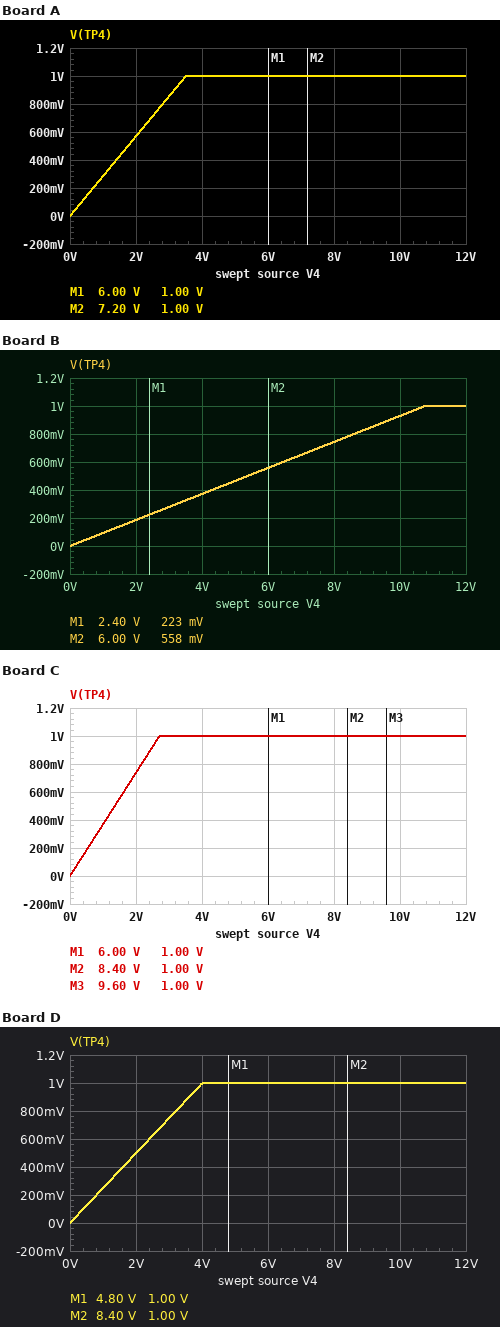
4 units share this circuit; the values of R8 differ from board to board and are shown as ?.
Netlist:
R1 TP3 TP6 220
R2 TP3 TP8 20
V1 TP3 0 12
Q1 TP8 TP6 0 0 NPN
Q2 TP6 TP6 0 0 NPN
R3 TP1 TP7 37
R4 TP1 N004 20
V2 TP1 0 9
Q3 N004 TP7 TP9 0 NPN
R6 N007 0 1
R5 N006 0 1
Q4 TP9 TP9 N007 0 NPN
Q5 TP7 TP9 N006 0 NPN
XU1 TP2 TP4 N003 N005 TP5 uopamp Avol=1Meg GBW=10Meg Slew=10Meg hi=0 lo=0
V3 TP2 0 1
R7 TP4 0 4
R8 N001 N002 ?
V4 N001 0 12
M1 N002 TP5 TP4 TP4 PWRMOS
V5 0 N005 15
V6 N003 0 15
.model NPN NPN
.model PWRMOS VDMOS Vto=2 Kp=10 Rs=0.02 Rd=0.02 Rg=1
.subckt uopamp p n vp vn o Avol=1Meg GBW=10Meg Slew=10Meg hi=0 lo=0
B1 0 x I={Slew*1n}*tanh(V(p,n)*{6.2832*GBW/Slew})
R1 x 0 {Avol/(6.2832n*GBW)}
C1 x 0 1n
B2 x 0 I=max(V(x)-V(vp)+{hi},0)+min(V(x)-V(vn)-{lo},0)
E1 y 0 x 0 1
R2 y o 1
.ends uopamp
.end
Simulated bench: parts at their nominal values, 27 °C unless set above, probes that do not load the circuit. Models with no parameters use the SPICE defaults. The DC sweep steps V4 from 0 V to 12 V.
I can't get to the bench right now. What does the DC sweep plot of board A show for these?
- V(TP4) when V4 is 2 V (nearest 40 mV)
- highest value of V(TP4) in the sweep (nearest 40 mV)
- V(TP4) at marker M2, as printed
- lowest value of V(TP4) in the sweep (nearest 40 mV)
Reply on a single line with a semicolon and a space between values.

560 mV; 1.00 V; 1.00 V; 0 V
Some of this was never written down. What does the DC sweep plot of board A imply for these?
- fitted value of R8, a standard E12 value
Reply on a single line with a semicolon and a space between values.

10 Ω
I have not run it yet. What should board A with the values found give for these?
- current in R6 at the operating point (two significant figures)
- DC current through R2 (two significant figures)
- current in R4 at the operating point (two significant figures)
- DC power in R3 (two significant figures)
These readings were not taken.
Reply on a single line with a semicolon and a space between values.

190 mA; 50 mA; 190 mA; 1.3 W
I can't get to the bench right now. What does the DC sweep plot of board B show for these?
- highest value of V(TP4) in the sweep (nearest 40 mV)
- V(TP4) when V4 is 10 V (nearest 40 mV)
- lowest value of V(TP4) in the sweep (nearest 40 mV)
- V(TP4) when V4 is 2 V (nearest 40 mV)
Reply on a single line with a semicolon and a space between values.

1.00 V; 920 mV; 0 V; 200 mV
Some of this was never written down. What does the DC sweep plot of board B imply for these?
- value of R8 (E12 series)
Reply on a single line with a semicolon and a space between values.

39 Ω
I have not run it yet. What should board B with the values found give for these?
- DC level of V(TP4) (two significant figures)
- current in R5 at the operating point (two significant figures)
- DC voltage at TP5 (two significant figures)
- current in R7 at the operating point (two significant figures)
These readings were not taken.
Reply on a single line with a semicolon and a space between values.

1.0 V; 190 mA; 3.2 V; 250 mA
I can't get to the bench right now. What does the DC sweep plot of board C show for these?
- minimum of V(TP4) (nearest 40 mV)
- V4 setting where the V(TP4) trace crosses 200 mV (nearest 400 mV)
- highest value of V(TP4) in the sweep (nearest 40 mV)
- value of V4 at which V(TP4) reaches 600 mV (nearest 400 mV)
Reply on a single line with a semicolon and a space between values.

0 V; 400 mV; 1.00 V; 1.6 V
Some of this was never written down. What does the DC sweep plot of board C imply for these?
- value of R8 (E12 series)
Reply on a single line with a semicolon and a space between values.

6.8 Ω
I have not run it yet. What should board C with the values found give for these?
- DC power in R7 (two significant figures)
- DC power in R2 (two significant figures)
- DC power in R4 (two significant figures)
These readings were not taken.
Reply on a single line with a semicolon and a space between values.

250 mW; 49 mW; 710 mW
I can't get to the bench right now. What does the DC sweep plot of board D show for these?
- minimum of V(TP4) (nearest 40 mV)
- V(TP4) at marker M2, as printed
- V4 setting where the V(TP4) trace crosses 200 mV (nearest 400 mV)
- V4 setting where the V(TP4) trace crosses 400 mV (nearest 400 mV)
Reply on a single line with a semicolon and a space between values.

0 V; 1.00 V; 800 mV; 1.6 V
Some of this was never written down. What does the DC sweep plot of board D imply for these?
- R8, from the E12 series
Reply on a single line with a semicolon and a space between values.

12 Ω
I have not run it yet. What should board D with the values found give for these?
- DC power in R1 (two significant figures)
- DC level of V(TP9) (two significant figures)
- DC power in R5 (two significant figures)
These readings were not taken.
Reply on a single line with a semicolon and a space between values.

560 mW; 1.1 V; 36 mW
